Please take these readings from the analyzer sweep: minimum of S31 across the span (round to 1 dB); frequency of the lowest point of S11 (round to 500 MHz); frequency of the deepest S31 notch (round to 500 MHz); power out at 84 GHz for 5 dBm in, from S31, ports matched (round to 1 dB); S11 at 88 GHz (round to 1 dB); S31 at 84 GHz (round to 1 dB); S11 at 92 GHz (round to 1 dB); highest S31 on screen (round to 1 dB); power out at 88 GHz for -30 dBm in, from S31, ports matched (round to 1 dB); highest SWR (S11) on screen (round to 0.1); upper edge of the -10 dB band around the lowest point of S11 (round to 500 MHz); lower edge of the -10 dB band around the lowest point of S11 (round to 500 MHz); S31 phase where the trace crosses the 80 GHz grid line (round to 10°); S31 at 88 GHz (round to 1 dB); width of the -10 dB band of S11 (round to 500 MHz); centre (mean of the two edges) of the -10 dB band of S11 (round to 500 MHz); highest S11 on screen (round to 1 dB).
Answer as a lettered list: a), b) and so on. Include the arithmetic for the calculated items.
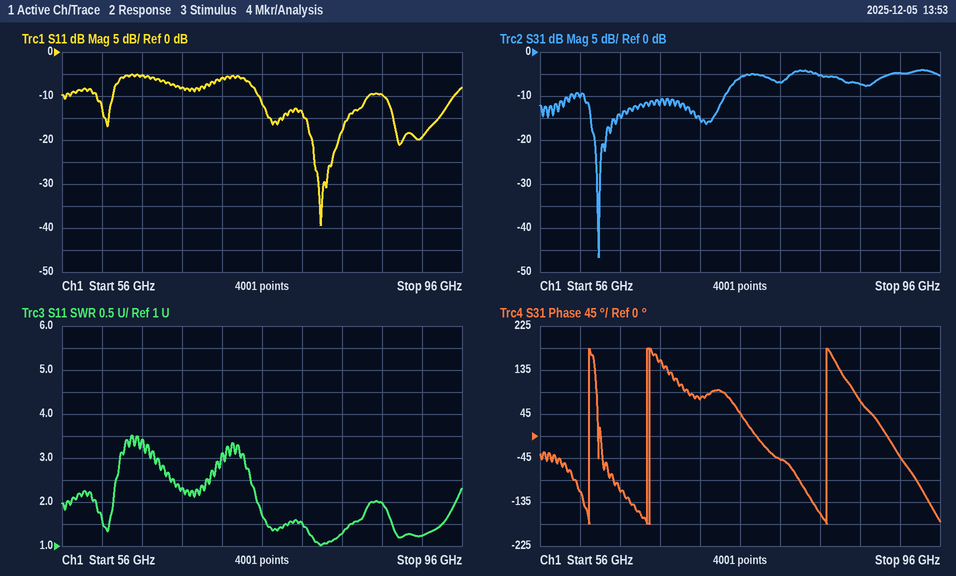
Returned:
a) -47 dB
b) 82.0 GHz
c) 62.0 GHz
d) 5 dBm + (-5 dB) = 0 dBm
e) -10 dB
f) -5 dB
g) -19 dB
h) -4 dB
i) -30 dBm + (-7 dB) = -37 dBm
j) 3.5
k) 86.5 GHz
l) 75.5 GHz
m) -50°
n) -7 dB
o) 86.5 GHz − 75.5 GHz = 11.0 GHz
p) 81.0 GHz
q) -5 dB
